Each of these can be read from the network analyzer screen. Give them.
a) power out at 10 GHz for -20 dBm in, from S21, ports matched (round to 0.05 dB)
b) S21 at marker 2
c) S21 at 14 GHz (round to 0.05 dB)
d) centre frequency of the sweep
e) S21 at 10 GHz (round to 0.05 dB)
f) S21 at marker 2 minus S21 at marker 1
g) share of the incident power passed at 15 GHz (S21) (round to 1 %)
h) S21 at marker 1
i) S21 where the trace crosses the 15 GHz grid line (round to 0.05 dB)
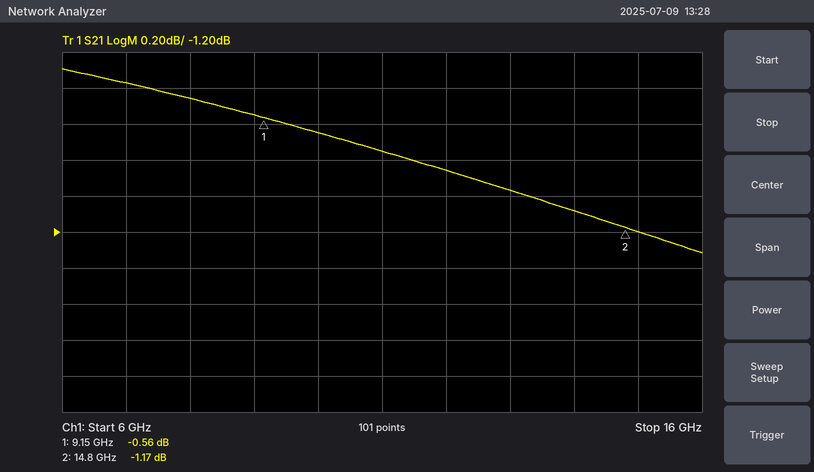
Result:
-20.65 dBm
-1.17 dB
-1.10 dB
11 GHz
-0.65 dB
-0.61 dB
76 %
-0.56 dB
-1.20 dB
